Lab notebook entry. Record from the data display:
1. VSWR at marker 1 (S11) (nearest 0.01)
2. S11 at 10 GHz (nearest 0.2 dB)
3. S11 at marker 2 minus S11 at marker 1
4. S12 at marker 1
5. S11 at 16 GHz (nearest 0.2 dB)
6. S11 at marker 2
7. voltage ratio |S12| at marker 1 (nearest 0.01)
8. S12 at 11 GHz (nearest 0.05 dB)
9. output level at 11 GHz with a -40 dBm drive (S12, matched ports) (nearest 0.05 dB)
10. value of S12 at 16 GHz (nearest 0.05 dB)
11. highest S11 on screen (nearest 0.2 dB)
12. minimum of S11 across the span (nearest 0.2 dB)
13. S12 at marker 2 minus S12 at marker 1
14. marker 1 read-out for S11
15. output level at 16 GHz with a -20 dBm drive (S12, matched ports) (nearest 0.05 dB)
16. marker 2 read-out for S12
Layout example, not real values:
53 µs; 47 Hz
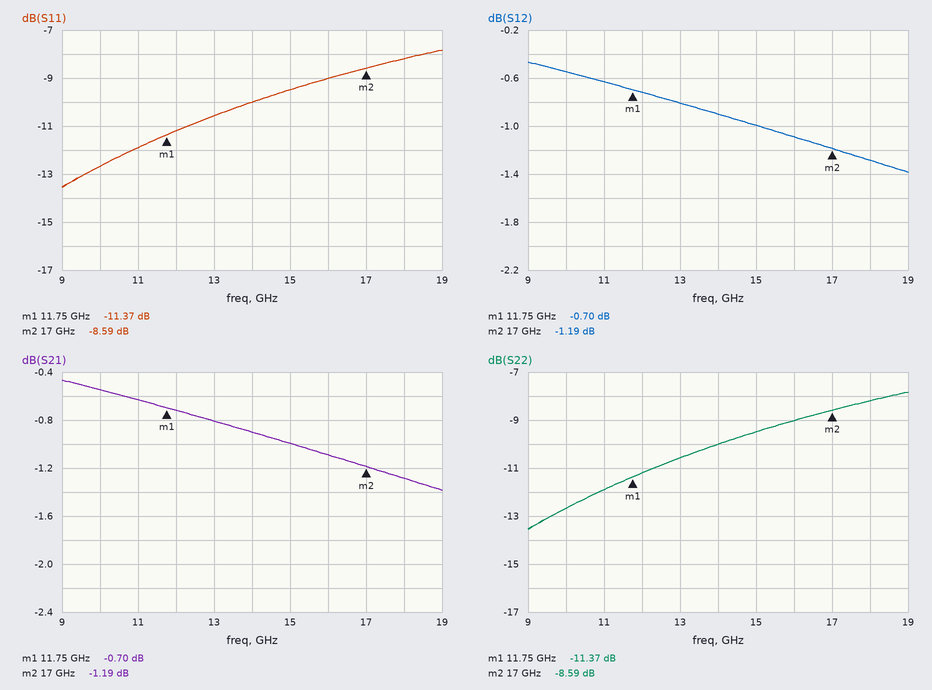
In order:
1.74; -12.6 dB; 2.78 dB; -0.70 dB; -9.0 dB; -8.59 dB; 0.92; -0.65 dB; -40.65 dBm; -1.10 dB; -7.8 dB; -13.6 dB; -0.49 dB; -11.37 dB; -21.10 dBm; -1.19 dB
